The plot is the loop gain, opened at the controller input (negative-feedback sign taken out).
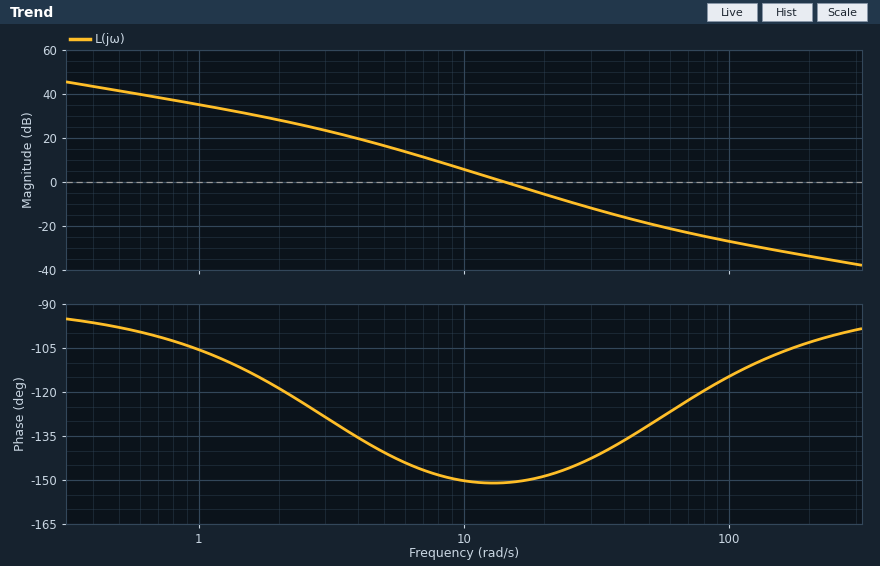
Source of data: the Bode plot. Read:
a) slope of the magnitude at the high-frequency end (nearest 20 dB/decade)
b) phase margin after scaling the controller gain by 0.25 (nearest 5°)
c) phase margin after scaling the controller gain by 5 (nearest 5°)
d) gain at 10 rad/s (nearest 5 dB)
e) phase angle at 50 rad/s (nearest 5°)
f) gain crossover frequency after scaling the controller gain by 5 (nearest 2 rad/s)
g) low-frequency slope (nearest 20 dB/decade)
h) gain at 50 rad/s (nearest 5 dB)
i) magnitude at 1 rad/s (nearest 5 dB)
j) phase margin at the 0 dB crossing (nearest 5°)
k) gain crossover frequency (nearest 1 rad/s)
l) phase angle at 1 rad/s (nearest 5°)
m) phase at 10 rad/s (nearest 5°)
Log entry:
-20 dB/decade
35°
40°
5 dB
-130°
34 rad/s
-20 dB/decade
-20 dB
35 dB
30°
14 rad/s
-105°
-150°
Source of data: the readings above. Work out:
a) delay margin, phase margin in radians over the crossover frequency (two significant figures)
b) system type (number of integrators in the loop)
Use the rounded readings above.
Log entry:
0.037 s
1
